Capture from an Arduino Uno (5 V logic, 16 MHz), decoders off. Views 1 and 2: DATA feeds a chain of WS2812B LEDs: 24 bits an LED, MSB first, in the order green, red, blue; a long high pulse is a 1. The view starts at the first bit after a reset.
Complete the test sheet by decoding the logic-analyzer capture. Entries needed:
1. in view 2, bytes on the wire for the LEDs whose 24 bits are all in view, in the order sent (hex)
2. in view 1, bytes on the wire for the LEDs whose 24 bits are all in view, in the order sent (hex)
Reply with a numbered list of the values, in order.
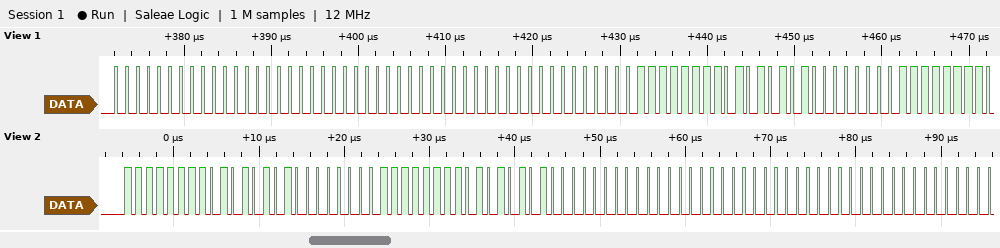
1. FF 55 00 FF 55 00 00 00 00
2. 00 00 00 00 00 00 FF 55 00
